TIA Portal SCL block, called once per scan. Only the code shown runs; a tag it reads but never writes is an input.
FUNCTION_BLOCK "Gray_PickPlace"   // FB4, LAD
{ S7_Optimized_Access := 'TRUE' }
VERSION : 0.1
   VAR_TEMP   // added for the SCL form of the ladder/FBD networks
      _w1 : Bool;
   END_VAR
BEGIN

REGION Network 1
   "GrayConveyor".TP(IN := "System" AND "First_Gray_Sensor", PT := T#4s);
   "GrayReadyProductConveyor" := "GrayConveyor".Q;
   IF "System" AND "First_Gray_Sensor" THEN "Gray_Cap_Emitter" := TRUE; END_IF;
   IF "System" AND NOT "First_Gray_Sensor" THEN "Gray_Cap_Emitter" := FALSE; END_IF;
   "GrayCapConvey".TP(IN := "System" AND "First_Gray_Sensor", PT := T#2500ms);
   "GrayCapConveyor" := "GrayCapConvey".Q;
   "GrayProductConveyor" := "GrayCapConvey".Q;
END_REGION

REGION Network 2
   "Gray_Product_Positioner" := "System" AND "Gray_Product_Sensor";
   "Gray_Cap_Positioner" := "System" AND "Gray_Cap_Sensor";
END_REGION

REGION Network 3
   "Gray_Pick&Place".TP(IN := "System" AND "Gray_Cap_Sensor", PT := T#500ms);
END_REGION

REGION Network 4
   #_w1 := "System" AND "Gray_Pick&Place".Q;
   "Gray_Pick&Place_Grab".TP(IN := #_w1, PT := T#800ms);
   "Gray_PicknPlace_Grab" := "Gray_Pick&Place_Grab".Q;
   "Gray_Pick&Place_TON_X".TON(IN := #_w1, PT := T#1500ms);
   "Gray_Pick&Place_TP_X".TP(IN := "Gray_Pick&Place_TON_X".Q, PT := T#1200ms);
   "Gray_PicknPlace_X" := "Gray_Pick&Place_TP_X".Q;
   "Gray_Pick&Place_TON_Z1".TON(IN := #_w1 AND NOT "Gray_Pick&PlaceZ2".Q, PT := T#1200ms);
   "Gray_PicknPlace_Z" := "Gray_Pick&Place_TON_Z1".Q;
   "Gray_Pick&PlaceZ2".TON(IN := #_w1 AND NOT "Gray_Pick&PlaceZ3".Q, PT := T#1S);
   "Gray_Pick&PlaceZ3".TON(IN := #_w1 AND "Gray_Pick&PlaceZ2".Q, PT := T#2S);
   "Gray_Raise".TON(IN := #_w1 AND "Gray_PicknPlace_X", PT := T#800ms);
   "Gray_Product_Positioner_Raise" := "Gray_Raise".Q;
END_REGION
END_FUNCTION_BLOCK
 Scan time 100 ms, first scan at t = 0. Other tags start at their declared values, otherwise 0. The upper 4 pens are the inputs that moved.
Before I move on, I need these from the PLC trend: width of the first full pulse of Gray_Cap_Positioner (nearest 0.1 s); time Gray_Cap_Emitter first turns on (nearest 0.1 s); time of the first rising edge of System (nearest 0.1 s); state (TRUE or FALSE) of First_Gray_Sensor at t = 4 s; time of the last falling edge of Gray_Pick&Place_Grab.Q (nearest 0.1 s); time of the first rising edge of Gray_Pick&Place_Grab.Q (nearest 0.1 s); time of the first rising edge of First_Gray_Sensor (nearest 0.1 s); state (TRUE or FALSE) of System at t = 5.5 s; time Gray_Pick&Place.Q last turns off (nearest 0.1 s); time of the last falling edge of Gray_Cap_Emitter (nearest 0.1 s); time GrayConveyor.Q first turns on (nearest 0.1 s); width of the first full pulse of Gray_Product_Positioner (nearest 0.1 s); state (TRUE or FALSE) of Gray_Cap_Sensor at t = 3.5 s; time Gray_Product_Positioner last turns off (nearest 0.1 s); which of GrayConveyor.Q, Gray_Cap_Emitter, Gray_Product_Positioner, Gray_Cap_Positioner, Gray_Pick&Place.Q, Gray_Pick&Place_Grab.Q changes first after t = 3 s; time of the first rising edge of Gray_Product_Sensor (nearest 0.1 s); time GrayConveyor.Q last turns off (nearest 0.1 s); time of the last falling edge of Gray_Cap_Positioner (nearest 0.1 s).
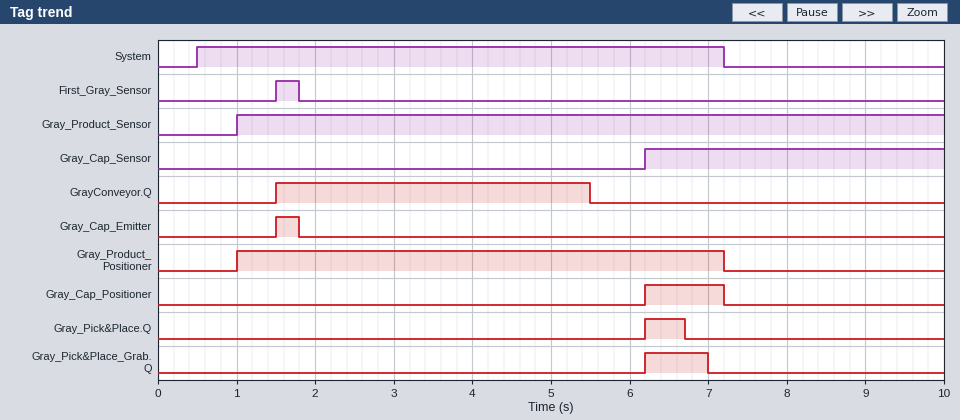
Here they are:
1.0 s
1.5 s
0.5 s
FALSE
7.0 s
6.2 s
1.5 s
TRUE
6.7 s
1.8 s
1.5 s
6.2 s
FALSE
7.2 s
GrayConveyor.Q
1.0 s
5.5 s
7.2 s
